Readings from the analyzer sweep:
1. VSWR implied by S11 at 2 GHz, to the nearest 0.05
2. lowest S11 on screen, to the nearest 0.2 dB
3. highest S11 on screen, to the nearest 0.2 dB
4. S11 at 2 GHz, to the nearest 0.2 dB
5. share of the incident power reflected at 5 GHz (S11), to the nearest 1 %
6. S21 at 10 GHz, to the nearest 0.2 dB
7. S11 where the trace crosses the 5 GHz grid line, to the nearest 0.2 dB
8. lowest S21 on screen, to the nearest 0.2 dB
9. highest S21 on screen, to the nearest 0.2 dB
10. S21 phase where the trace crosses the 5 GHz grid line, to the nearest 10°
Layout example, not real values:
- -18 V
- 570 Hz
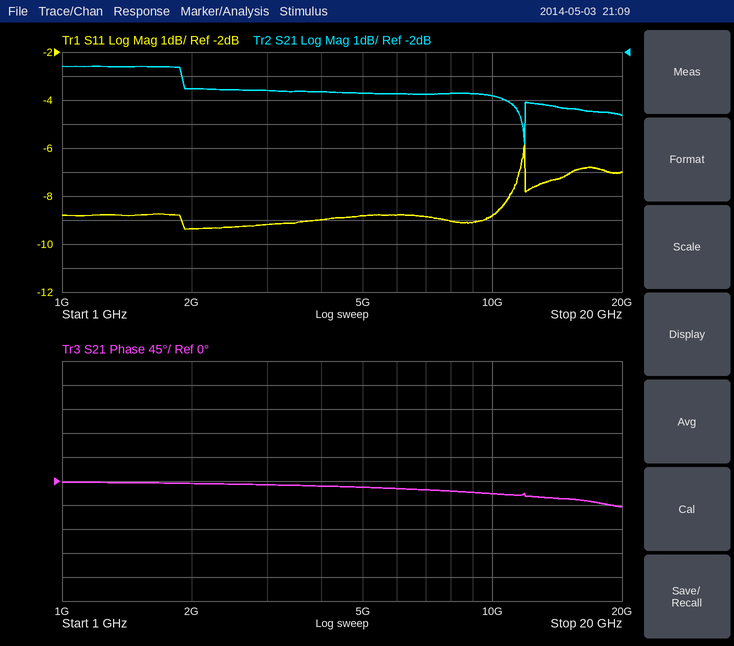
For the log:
- 2.05
- -9.4 dB
- -5.8 dB
- -9.4 dB
- 13 %
- -3.8 dB
- -8.8 dB
- -5.8 dB
- -2.6 dB
- -10°
